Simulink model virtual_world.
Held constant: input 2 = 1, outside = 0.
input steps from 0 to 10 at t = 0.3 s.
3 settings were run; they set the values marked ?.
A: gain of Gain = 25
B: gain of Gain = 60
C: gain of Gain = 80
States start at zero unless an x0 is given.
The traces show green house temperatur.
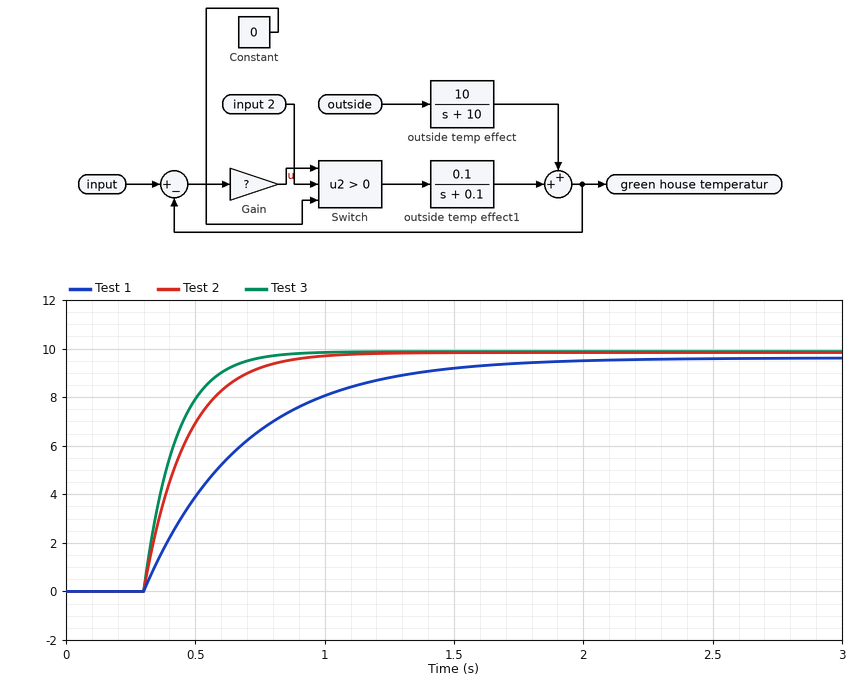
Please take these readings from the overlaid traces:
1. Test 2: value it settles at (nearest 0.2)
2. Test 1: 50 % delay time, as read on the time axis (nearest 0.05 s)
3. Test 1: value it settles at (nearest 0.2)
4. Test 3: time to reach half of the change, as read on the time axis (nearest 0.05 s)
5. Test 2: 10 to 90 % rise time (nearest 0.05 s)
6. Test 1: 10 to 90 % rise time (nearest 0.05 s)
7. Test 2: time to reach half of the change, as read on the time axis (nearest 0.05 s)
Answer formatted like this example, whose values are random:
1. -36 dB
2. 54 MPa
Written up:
1. 9.8
2. 0.55 s
3. 9.6
4. 0.40 s
5. 0.35 s
6. 0.85 s
7. 0.40 s
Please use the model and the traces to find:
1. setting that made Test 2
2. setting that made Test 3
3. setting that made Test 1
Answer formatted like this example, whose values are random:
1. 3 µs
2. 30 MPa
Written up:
1. B
2. C
3. A
